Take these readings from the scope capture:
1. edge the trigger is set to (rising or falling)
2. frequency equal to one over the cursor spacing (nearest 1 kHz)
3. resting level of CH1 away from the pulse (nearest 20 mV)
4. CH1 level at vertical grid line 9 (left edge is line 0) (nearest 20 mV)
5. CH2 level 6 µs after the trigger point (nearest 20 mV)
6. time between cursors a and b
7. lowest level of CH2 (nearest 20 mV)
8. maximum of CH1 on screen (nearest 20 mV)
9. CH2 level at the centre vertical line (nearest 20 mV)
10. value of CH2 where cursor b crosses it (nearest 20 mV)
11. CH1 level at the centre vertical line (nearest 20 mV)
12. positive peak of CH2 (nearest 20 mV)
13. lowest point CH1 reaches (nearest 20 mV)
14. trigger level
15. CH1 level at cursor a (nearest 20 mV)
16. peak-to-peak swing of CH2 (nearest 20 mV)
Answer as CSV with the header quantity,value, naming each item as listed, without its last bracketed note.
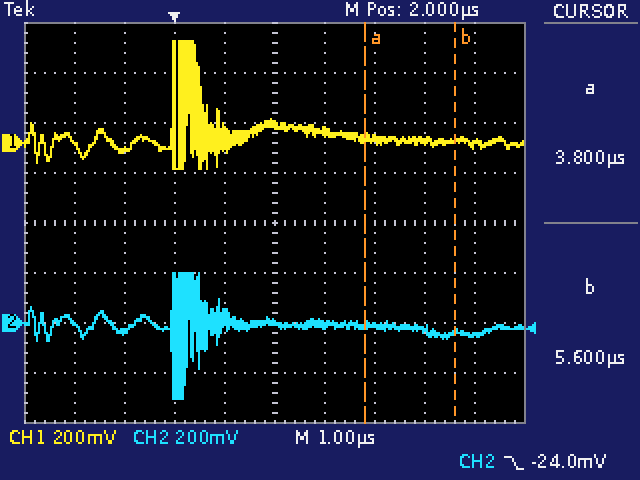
quantity,value
edge the trigger is set to,falling
frequency equal to one over the cursor spacing,556 kHz
resting level of CH1 away from the pulse,20 mV
CH1 level at vertical grid line 9 (left edge is line 0),0 mV
CH2 level 6 µs after the trigger point,-40 mV
time between cursors a and b,1.8 µs
lowest level of CH2,-300 mV
maximum of CH1 on screen,400 mV
CH2 level at the centre vertical line,0 mV
value of CH2 where cursor b crosses it,-40 mV
CH1 level at the centre vertical line,80 mV
positive peak of CH2,200 mV
lowest point CH1 reaches,-100 mV
trigger level,-24.0 mV
CH1 level at cursor a,20 mV
peak-to-peak swing of CH2,500 mV
